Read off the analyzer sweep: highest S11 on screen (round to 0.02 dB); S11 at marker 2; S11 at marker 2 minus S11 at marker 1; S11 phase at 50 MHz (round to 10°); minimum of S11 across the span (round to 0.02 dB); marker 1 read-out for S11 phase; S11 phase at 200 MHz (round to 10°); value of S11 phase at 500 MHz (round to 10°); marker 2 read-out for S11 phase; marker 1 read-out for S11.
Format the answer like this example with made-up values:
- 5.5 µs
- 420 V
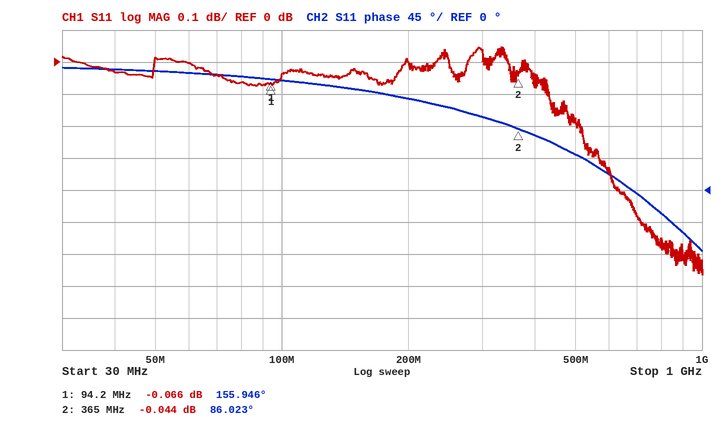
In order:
- 0.04 dB
- -0.044 dB
- 0.022 dB
- 170°
- -0.66 dB
- 155.946°
- 130°
- 50°
- 86.023°
- -0.066 dB
